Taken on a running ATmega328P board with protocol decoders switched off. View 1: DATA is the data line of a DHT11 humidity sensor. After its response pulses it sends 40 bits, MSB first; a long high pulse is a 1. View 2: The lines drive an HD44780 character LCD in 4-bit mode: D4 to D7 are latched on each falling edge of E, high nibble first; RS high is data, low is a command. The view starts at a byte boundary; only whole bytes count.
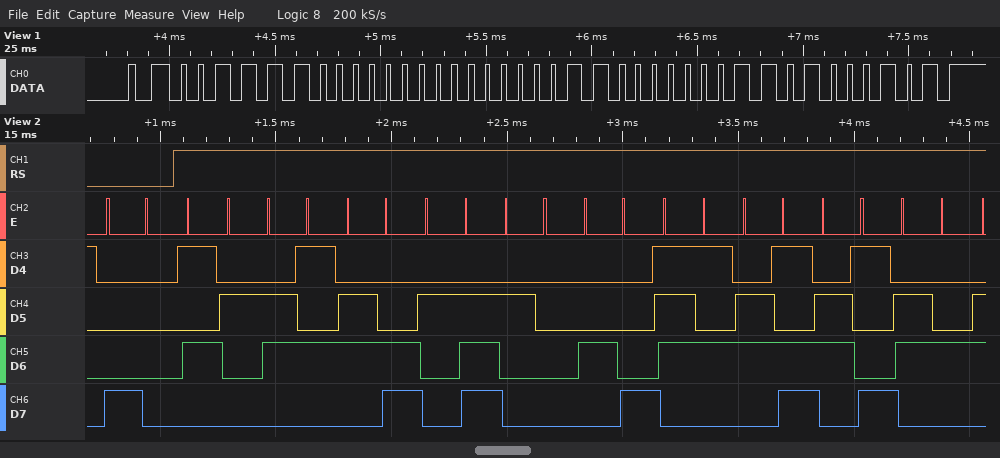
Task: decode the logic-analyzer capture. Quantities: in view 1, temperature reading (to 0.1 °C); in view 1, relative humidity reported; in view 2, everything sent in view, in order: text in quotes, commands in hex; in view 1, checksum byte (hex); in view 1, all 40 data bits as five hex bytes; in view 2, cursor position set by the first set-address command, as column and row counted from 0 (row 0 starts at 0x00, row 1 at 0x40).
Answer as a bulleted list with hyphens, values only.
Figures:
- 6.3 °C
- 60 %
- 0x80 "Rel. Humid"
- 0x45
- 3C 00 06 03 45
- column 0, row 0
